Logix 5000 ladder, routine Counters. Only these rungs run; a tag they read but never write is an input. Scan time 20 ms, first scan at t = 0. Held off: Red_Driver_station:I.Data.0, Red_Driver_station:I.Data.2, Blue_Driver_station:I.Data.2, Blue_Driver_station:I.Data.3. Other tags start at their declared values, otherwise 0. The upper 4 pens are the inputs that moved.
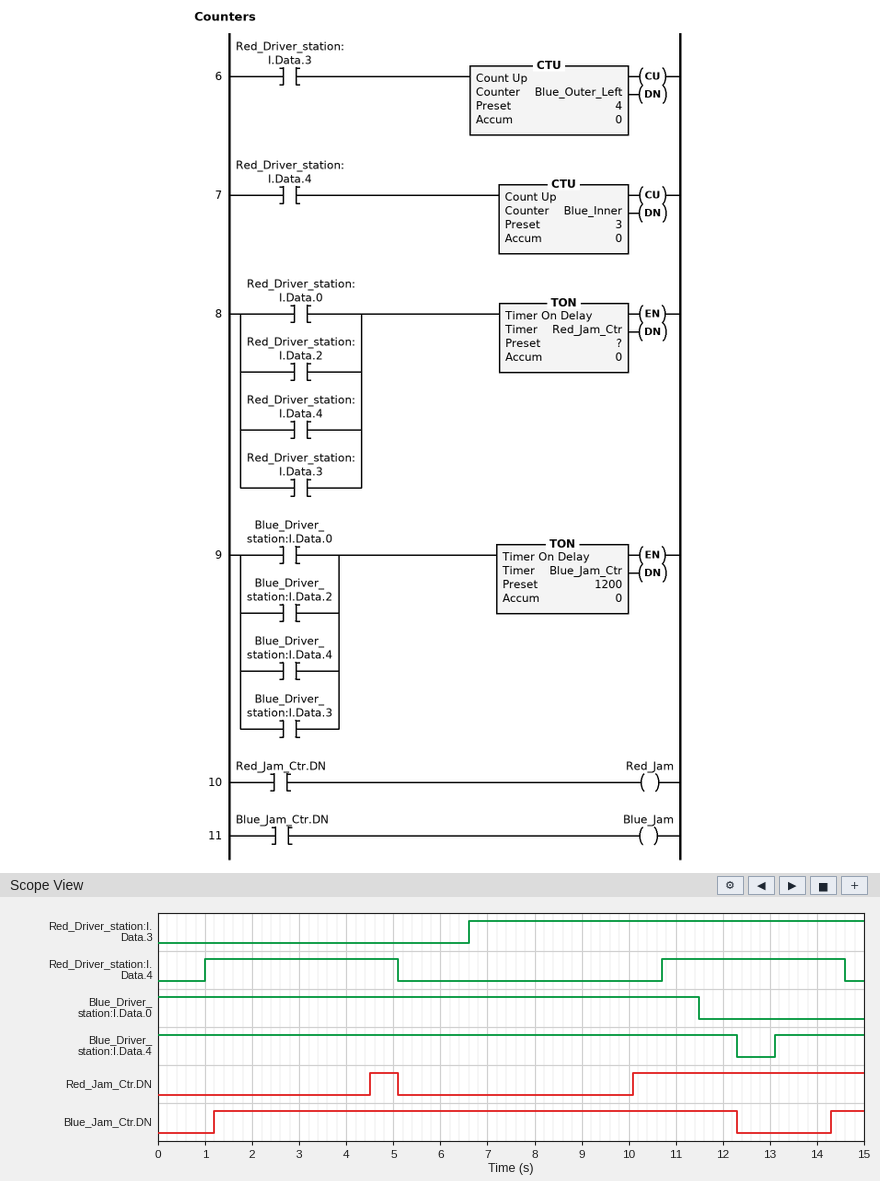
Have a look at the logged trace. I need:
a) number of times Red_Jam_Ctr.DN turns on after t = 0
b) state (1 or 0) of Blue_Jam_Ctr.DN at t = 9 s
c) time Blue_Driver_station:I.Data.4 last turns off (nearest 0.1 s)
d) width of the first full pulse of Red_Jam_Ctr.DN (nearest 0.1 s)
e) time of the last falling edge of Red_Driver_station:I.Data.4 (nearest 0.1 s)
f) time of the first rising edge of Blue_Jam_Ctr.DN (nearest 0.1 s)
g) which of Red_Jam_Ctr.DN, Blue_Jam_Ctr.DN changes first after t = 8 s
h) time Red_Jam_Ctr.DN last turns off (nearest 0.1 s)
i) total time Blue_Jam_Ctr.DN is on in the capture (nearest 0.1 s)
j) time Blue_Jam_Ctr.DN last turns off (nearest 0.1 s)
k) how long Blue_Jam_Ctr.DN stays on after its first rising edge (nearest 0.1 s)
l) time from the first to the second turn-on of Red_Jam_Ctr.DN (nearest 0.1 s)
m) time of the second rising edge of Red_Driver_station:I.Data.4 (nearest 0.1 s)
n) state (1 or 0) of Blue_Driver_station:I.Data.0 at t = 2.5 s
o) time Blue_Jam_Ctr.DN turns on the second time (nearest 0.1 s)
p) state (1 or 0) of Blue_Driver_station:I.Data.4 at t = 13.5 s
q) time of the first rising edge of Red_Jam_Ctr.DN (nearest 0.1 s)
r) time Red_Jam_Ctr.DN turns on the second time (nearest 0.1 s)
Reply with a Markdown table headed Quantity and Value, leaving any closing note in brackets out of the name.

| Quantity | Value |
|---|---|
| number of times Red_Jam_Ctr.DN turns on after t = 0 | 2 |
| state (1 or 0) of Blue_Jam_Ctr.DN at t = 9 s | 1 |
| time Blue_Driver_station:I.Data.4 last turns off | 12.3 s |
| width of the first full pulse of Red_Jam_Ctr.DN | 0.6 s |
| time of the last falling edge of Red_Driver_station:I.Data.4 | 14.6 s |
| time of the first rising edge of Blue_Jam_Ctr.DN | 1.2 s |
| which of Red_Jam_Ctr.DN, Blue_Jam_Ctr.DN changes first after t = 8 s | Red_Jam_Ctr.DN |
| time Red_Jam_Ctr.DN last turns off | 5.1 s |
| total time Blue_Jam_Ctr.DN is on in the capture | 11.8 s |
| time Blue_Jam_Ctr.DN last turns off | 12.3 s |
| how long Blue_Jam_Ctr.DN stays on after its first rising edge | 11.1 s |
| time from the first to the second turn-on of Red_Jam_Ctr.DN | 5.6 s |
| time of the second rising edge of Red_Driver_station:I.Data.4 | 10.7 s |
| state (1 or 0) of Blue_Driver_station:I.Data.0 at t = 2.5 s | 1 |
| time Blue_Jam_Ctr.DN turns on the second time | 14.3 s |
| state (1 or 0) of Blue_Driver_station:I.Data.4 at t = 13.5 s | 1 |
| time of the first rising edge of Red_Jam_Ctr.DN | 4.5 s |
| time Red_Jam_Ctr.DN turns on the second time | 10.1 s |
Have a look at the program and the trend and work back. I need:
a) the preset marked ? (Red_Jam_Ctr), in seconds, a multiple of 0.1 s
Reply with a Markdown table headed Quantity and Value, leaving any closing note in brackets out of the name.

| Quantity | Value |
|---|---|
| the preset marked ? (Red_Jam_Ctr), in seconds, a multiple of 0.1 s | 3.5 s |
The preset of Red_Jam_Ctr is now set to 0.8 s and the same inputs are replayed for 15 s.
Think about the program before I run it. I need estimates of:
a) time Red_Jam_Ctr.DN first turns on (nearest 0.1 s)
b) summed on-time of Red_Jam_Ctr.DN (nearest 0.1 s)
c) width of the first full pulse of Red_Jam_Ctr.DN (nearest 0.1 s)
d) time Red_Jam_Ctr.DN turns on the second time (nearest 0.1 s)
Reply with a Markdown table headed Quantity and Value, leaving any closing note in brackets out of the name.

| Quantity | Value |
|---|---|
| time Red_Jam_Ctr.DN first turns on | 1.8 s |
| summed on-time of Red_Jam_Ctr.DN | 10.9 s |
| width of the first full pulse of Red_Jam_Ctr.DN | 3.3 s |
| time Red_Jam_Ctr.DN turns on the second time | 7.4 s |
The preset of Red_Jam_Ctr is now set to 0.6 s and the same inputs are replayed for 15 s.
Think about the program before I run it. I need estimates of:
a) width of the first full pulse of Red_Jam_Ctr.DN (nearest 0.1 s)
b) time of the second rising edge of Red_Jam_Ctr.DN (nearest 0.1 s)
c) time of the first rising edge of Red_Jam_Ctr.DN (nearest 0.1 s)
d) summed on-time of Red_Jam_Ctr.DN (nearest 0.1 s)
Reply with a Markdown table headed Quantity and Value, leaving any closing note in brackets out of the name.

| Quantity | Value |
|---|---|
| width of the first full pulse of Red_Jam_Ctr.DN | 3.5 s |
| time of the second rising edge of Red_Jam_Ctr.DN | 7.2 s |
| time of the first rising edge of Red_Jam_Ctr.DN | 1.6 s |
| summed on-time of Red_Jam_Ctr.DN | 11.3 s |
